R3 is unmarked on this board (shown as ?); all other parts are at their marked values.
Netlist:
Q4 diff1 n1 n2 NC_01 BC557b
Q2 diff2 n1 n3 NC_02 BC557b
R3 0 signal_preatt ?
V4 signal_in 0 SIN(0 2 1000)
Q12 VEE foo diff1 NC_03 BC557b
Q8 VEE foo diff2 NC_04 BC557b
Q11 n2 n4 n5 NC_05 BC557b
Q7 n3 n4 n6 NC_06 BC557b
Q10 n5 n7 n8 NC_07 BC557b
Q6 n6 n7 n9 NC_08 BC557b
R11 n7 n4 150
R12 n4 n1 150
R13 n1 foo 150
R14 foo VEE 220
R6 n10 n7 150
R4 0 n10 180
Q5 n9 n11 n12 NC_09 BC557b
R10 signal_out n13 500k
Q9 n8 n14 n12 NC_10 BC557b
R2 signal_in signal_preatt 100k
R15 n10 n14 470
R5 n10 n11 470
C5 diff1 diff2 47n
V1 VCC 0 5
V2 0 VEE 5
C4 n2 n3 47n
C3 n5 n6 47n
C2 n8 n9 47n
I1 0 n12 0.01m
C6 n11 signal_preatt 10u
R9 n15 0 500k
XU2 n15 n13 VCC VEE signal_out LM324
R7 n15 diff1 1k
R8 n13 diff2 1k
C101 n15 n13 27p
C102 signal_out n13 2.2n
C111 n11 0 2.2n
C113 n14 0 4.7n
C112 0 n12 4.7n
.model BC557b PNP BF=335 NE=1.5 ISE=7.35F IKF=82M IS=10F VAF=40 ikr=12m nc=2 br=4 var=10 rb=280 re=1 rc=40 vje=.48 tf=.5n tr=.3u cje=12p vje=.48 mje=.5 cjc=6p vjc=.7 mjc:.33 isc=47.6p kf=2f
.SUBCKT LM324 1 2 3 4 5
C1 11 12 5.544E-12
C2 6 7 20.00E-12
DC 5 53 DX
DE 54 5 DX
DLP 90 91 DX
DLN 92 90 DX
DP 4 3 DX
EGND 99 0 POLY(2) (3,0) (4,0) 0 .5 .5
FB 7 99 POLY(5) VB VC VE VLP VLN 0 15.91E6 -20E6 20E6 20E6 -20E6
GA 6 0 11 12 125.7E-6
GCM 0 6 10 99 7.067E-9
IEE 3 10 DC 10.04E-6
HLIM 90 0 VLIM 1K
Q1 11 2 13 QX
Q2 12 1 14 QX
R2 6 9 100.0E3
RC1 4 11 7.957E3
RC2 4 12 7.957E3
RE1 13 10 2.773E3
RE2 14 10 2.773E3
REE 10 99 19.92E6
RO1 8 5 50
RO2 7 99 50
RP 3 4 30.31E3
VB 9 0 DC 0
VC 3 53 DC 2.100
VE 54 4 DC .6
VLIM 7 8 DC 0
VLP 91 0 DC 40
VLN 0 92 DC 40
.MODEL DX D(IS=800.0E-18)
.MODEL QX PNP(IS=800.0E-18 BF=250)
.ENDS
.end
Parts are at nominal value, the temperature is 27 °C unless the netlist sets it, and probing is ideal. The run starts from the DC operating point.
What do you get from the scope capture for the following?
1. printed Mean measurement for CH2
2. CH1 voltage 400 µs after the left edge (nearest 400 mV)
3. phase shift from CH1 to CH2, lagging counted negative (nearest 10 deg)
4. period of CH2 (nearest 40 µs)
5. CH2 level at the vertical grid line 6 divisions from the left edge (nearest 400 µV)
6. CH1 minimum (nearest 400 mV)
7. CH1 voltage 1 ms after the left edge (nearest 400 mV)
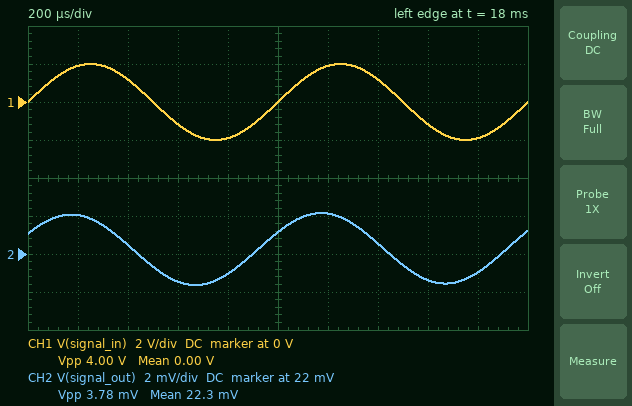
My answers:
22.3 mV
1.2 V
30 deg
1.00 ms
24.0 mV
-2.0 V
0 V
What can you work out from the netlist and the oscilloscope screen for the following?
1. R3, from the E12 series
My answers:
1.2 kΩ
